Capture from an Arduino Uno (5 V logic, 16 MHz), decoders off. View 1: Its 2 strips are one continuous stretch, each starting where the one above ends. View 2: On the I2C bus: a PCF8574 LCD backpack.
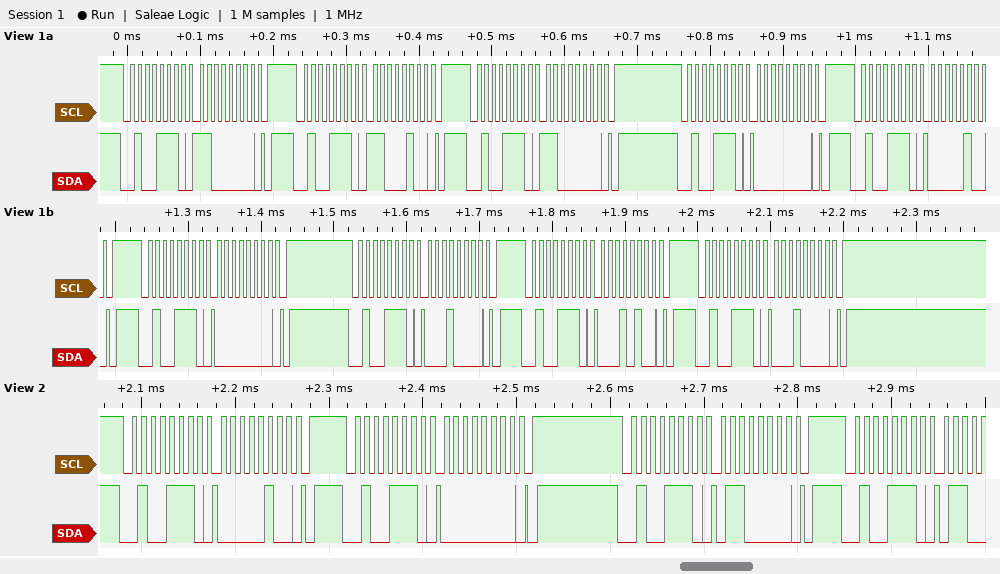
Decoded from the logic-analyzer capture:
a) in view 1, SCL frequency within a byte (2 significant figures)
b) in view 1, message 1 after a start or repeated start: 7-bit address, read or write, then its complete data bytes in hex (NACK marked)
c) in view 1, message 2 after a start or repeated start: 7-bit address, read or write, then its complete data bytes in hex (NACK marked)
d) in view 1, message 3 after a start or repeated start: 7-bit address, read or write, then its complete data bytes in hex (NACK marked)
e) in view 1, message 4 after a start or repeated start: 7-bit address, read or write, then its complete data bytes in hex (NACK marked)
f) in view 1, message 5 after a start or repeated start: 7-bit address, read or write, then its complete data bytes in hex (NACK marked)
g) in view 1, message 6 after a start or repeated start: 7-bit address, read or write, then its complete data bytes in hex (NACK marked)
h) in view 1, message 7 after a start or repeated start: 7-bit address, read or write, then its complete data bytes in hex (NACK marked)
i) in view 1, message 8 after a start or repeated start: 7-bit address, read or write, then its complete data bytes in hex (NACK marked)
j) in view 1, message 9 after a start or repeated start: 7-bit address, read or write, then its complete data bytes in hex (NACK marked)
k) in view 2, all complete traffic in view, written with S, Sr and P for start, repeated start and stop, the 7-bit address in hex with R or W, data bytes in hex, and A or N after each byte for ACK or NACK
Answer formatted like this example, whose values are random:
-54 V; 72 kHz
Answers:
100 kHz; 0x27 write: C0; 0x27 write: C4; 0x27 write: C0; 0x27 write: 00; 0x27 write: 04; 0x27 write: 00; 0x27 write: 10; 0x27 write: 14; 0x27 write: 10; S 27W A 04 A P S 27W A 00 A P S 27W A 60 A P S 27W A
